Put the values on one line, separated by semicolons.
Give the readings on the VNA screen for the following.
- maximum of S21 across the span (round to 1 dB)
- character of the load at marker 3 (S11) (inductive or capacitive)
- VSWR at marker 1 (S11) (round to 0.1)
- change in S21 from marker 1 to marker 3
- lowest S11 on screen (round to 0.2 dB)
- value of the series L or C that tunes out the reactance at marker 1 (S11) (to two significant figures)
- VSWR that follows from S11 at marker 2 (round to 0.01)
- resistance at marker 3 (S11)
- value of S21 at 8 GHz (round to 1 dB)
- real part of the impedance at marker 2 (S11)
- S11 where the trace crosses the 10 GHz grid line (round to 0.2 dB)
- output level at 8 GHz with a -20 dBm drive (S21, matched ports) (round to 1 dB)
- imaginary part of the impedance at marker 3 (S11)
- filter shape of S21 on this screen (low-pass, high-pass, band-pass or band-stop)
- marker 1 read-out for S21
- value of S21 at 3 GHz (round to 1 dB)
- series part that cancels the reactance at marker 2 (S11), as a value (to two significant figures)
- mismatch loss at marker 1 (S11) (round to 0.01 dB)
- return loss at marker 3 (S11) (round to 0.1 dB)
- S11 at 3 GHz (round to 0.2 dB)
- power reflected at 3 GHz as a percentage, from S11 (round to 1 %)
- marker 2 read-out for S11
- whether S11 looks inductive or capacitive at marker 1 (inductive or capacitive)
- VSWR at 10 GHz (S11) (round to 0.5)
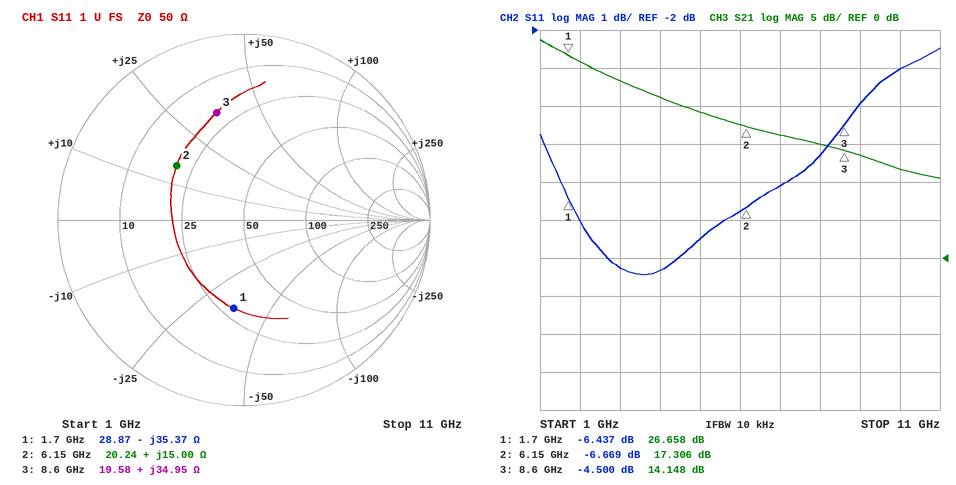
29 dB; inductive; 2.8; -12.510 dB; -8.4 dB; 3.3 nH; 2.73; 19.58 Ω; 15 dB; 20.24 Ω; -3.0 dB; -5 dBm; +34.95 Ω; low-pass; 26.658 dB; 23 dB; 1.7 pF; 1.12 dB; 4.5 dB; -8.2 dB; 15 %; -6.669 dB; capacitive; 6.0
